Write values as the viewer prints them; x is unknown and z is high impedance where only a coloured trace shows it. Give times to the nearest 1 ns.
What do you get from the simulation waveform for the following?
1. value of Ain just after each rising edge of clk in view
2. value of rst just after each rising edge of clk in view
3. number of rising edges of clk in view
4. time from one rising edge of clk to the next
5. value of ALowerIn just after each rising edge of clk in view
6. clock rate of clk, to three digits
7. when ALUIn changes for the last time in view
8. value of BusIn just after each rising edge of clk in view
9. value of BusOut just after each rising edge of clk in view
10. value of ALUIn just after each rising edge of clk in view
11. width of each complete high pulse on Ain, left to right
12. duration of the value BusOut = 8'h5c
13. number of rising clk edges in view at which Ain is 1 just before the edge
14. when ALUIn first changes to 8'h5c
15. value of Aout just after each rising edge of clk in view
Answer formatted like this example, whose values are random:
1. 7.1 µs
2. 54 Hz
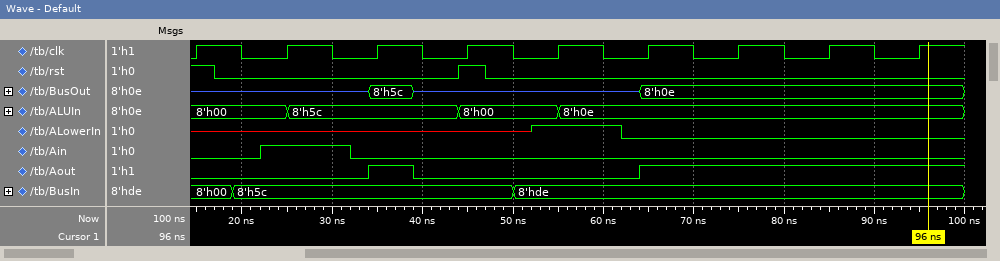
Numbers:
1. 0 1 0 0 0 0 0 0 0
2. 1 0 0 1 0 0 0 0 0
3. 9
4. 10 ns
5. x x x x 1 0 0 0 0
6. 100 MHz
7. 55 ns
8. 8'h00, 8'h5c, 8'h5c, 8'h5c, 8'hde, 8'hde, 8'hde, 8'hde, 8'hde
9. z, z, 8'h5c, z, z, 8'h0e, 8'h0e, 8'h0e, 8'h0e
10. 8'h00, 8'h5c, 8'h5c, 8'h00, 8'h0e, 8'h0e, 8'h0e, 8'h0e, 8'h0e
11. 10 ns
12. 5 ns
13. 1
14. 25 ns
15. 0 0 1 0 0 1 1 1 1
